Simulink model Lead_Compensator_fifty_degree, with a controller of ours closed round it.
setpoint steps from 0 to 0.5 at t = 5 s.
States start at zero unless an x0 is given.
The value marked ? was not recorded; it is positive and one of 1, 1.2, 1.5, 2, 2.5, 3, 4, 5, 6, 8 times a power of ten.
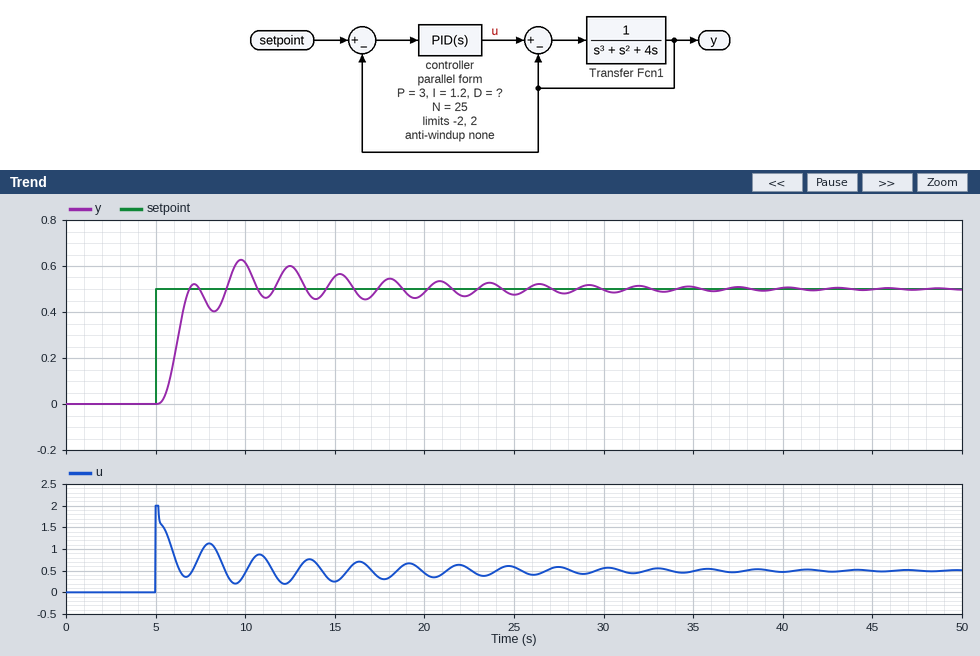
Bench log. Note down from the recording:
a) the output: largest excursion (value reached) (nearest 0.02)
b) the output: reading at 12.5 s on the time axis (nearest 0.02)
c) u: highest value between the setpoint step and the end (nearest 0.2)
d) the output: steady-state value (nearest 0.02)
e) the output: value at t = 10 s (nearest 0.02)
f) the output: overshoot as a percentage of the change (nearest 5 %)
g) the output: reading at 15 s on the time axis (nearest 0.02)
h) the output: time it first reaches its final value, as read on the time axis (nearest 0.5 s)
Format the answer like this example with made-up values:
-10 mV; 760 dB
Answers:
0.62; 0.60; 2.0; 0.50; 0.62; 25 %; 0.56; 7.0 s
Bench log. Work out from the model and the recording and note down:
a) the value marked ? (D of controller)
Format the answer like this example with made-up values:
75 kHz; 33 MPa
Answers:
1.5
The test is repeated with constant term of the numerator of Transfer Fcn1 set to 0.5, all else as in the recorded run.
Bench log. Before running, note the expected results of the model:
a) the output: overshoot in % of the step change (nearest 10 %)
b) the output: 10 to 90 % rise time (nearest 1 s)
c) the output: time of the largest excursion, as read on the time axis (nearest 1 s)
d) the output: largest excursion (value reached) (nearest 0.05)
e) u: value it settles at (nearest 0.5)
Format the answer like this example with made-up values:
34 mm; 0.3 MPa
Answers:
20 %; 3 s; 13 s; 0.60; 0.5
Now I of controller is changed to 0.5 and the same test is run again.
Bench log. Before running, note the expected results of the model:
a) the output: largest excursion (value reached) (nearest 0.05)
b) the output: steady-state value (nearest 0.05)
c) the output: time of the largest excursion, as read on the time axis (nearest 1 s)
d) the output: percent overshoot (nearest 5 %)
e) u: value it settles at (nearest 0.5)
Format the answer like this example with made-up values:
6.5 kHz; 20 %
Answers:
0.55; 0.50; 12 s; 10 %; 0.5
